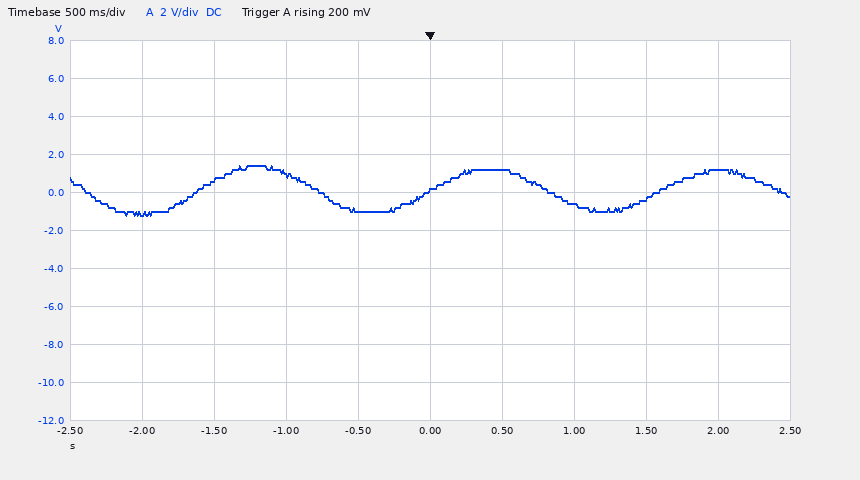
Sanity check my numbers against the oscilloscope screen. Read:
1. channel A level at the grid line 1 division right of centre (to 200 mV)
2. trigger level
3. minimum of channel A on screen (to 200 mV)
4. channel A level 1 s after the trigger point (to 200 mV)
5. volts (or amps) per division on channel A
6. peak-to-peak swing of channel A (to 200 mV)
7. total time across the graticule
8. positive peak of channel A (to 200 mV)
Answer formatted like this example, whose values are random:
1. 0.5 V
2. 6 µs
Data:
1. 1.2 V
2. 200 mV
3. -1.2 V
4. -600 mV
5. 2 V
6. 2.6 V
7. 5 s
8. 1.4 V
